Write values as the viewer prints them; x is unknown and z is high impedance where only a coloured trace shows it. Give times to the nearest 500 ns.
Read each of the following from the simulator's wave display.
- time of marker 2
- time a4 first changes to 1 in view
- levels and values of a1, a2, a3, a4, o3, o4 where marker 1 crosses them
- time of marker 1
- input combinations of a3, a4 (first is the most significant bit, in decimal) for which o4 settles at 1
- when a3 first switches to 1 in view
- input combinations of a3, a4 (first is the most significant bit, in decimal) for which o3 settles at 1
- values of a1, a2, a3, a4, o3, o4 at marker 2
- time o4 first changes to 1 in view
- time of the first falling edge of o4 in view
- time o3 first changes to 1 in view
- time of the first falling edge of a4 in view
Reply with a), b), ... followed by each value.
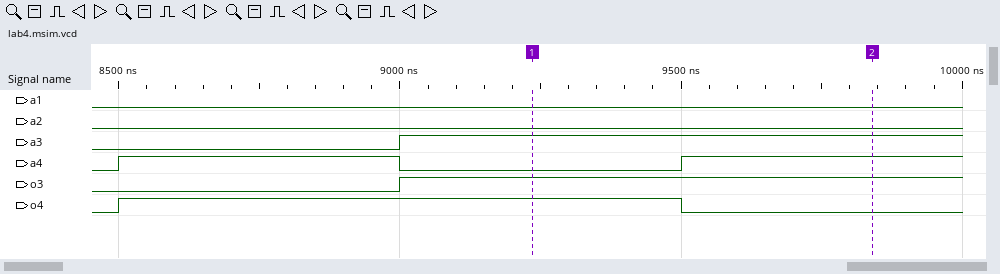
a) 10000 ns
b) 8500 ns
c) a1=0, a2=0, a3=1, a4=0, o3=1, o4=1
d) 9000 ns
e) 1, 2
f) 9000 ns
g) 2, 3
h) a1=0, a2=0, a3=1, a4=1, o3=1, o4=0
i) 8500 ns
j) 9500 ns
k) 9000 ns
l) 9000 ns
